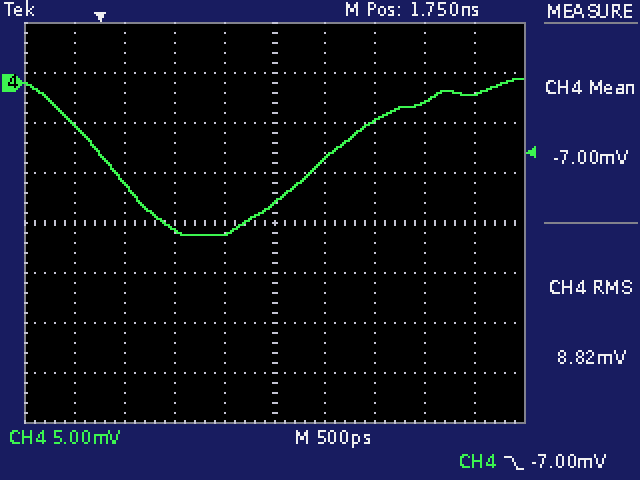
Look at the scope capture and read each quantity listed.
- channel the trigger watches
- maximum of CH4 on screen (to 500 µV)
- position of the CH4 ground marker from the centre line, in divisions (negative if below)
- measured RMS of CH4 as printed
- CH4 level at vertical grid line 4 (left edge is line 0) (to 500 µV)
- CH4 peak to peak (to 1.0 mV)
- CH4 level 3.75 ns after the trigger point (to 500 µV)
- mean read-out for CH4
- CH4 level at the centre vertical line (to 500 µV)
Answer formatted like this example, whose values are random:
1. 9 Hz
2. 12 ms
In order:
1. CH4
2. 500 µV
3. +2.8 div
4. 8.82 mV
5. -15.0 mV
6. 16.0 mV
7. -1.0 mV
8. -7.00 mV
9. -12.0 mV
